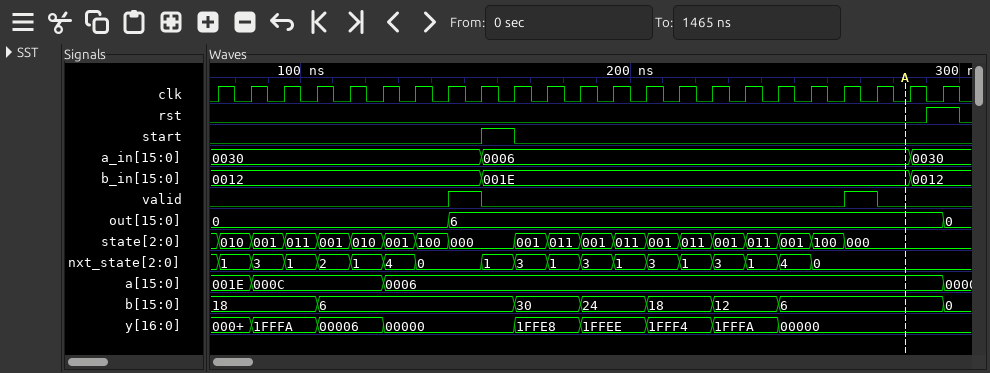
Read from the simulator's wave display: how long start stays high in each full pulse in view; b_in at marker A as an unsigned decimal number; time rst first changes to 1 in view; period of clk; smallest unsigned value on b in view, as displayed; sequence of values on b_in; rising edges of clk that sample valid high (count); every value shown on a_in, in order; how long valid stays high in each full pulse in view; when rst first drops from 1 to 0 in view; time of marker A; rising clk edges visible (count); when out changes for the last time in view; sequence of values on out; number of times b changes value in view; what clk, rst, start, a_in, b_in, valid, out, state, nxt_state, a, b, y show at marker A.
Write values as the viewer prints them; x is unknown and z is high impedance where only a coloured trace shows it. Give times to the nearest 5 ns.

10 ns
30
290 ns
10 ns
0
0012, 001E, 0012
2
0030, 0006, 0030
10 ns, 10 ns
300 ns
285 ns
23
295 ns
0, 6, 0
7
clk=0, rst=0, start=0, a_in=0006, b_in=001E, valid=0, out=6, state=000, nxt_state=0, a=0006, b=6, y=00000
